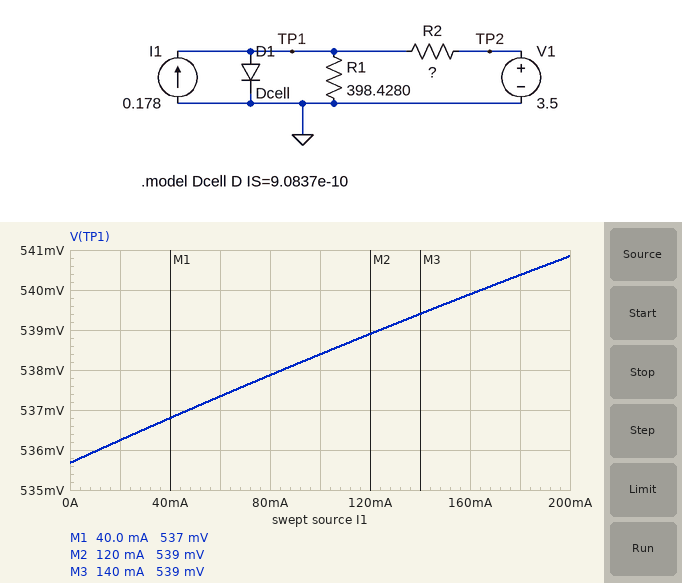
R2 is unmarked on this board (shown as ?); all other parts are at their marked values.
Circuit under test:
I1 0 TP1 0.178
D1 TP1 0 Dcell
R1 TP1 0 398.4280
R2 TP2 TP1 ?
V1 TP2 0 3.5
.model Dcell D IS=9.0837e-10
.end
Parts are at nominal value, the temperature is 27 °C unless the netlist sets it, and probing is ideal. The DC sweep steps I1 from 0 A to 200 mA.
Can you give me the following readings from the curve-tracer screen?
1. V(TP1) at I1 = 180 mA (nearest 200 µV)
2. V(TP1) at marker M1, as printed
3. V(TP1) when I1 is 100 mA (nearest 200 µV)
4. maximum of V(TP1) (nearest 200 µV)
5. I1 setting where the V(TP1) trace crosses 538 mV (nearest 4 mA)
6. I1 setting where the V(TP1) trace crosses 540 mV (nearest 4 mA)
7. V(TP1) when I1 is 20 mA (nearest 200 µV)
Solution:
540.4 mV
537 mV
538.4 mV
540.8 mV
84 mA
164 mA
536.2 mV
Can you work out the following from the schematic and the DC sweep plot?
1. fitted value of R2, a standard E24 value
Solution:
3.3 Ω
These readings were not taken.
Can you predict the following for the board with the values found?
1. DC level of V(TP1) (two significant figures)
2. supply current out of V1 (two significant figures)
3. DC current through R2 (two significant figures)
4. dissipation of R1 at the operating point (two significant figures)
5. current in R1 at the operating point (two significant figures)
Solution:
540 mV
900 mA
900 mA
730 µW
1.4 mA
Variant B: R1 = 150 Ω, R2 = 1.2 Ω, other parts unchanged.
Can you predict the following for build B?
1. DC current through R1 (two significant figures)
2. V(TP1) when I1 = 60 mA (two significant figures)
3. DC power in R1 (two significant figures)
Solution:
3.8 mA
560 mV
2.1 mW
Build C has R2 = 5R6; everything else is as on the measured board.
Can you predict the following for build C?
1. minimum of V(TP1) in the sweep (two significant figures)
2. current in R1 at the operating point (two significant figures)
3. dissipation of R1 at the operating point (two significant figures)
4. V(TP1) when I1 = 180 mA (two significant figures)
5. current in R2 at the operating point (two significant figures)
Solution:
520 mV
1.3 mA
700 µW
530 mV
530 mA
